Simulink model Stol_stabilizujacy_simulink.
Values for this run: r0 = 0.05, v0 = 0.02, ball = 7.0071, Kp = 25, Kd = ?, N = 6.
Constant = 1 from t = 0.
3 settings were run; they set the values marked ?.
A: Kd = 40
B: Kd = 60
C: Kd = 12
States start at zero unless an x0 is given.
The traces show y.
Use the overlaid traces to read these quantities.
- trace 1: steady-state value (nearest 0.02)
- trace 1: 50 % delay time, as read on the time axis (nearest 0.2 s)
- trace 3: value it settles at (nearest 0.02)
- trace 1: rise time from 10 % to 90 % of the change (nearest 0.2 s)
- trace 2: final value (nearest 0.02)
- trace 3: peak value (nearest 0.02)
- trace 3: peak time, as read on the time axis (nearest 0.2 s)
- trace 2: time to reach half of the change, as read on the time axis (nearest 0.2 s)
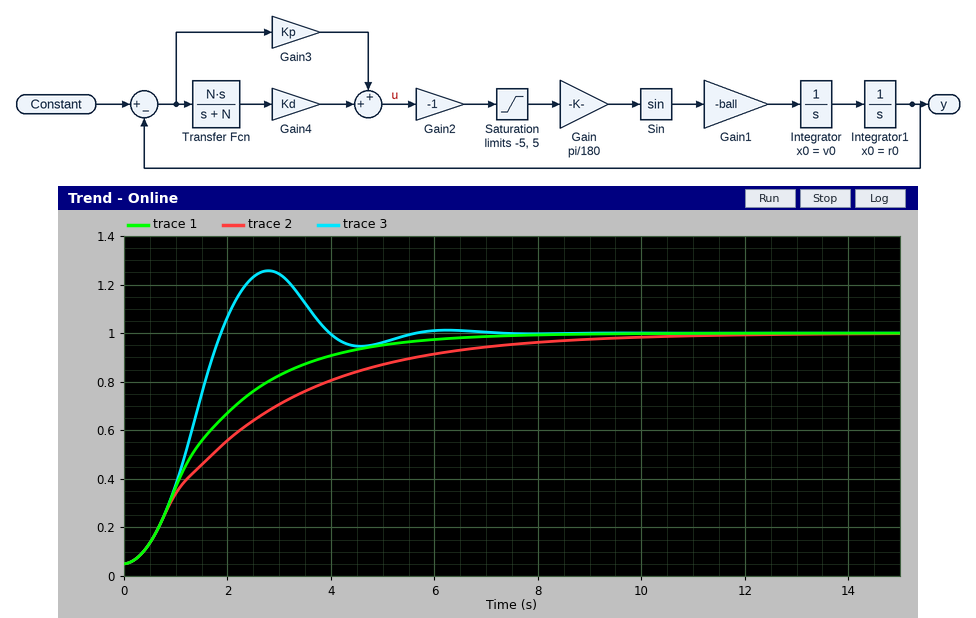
1.00
1.4 s
1.00
3.4 s
1.00
1.26
2.8 s
1.8 s
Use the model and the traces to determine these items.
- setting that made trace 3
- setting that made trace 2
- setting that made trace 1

C
B
A
